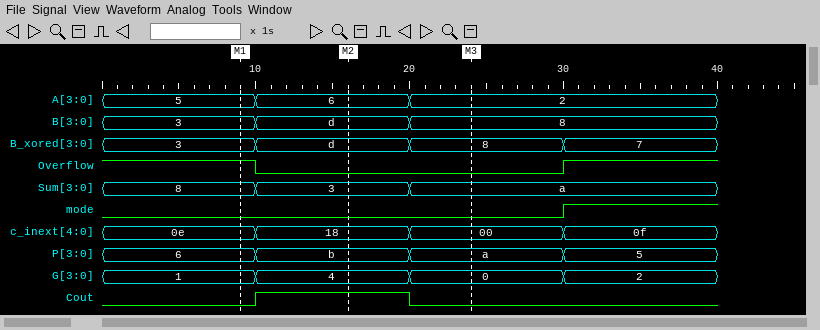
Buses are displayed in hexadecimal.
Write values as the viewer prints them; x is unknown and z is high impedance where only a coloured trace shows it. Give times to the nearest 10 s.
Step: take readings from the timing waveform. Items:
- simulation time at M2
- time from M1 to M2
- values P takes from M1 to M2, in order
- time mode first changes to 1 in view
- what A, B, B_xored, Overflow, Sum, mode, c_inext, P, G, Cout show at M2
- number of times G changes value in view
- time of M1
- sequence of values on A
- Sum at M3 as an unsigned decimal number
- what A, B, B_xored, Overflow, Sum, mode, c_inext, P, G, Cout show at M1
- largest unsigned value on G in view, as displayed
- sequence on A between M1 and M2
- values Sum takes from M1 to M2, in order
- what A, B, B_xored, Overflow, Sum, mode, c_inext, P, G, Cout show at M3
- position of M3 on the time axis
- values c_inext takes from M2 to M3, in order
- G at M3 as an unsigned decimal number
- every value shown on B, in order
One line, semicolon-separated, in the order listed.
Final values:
20 s; 10 s; 6, b; 30 s; A=6, B=d, B_xored=d, Overflow=0, Sum=3, mode=0, c_inext=18, P=b, G=4, Cout=1; 3; 10 s; 5, 6, 2; 10; A=5, B=3, B_xored=3, Overflow=1, Sum=8, mode=0, c_inext=0e, P=6, G=1, Cout=0; 4; 5, 6; 8, 3; A=2, B=8, B_xored=8, Overflow=0, Sum=a, mode=0, c_inext=00, P=a, G=0, Cout=0; 20 s; 18, 00; 0; 3, d, 8
